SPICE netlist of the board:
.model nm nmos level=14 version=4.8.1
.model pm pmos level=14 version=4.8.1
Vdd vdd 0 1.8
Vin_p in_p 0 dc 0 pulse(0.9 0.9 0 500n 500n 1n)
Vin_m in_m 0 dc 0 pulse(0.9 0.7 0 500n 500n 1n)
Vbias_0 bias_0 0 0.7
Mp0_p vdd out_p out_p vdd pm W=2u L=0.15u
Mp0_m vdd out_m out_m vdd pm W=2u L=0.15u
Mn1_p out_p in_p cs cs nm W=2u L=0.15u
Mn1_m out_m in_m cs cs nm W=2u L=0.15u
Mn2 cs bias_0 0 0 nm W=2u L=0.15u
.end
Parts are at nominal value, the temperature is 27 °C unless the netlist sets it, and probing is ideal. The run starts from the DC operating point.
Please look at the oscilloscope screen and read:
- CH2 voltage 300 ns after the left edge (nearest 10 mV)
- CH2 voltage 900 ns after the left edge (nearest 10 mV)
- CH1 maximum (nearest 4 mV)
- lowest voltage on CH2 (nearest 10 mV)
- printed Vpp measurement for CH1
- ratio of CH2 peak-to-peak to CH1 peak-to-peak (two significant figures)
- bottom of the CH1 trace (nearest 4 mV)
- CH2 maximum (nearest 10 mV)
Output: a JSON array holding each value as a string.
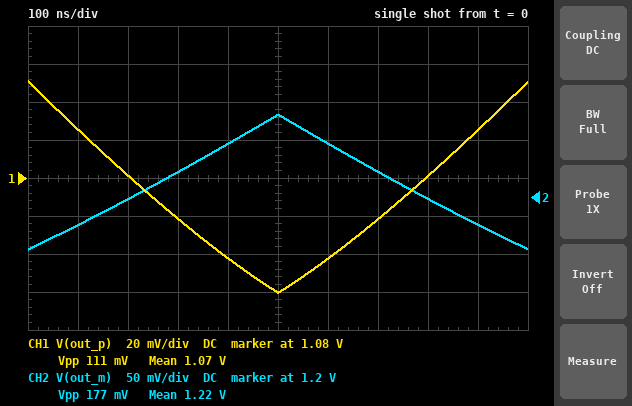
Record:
["1.23 V", "1.16 V", "1.132 V", "1.13 V", "111 mV", "1.6", "1.020 V", "1.31 V"]
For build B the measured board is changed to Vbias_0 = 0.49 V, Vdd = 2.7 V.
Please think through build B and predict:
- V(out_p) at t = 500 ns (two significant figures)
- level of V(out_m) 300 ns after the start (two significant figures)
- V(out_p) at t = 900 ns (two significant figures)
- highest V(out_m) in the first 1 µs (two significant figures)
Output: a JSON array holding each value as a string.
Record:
["2.1 V", "2.3 V", "2.2 V", "2.4 V"]
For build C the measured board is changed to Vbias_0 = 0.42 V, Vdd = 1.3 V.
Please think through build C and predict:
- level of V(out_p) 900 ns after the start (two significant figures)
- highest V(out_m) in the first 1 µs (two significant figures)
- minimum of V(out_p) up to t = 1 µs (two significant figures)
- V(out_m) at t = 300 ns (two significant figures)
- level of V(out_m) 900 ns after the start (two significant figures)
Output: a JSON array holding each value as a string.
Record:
["840 mV", "1.0 V", "820 mV", "950 mV", "890 mV"]
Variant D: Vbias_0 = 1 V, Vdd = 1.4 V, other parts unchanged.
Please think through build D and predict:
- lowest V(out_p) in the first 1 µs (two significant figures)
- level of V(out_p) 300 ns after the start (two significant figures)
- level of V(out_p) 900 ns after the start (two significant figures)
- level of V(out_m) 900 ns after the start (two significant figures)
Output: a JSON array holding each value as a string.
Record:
["540 mV", "560 mV", "590 mV", "630 mV"]
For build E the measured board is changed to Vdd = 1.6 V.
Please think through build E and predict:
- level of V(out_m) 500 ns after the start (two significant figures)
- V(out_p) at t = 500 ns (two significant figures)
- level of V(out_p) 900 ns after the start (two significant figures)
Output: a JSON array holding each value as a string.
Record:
["1.1 V", "830 mV", "910 mV"]
